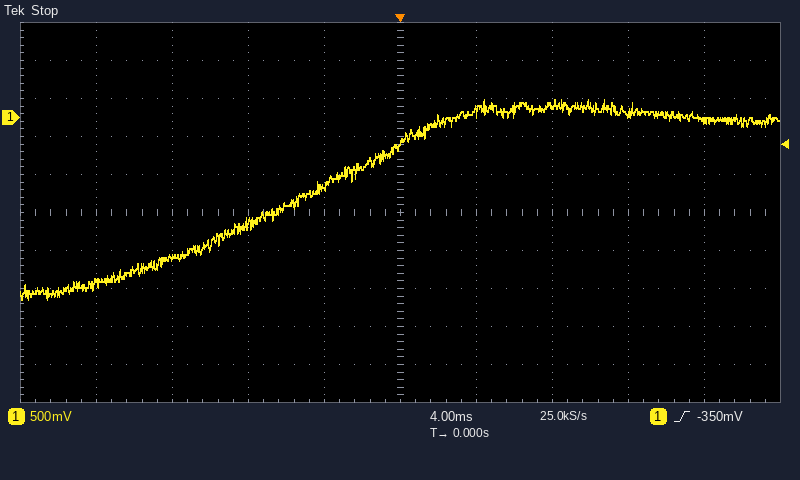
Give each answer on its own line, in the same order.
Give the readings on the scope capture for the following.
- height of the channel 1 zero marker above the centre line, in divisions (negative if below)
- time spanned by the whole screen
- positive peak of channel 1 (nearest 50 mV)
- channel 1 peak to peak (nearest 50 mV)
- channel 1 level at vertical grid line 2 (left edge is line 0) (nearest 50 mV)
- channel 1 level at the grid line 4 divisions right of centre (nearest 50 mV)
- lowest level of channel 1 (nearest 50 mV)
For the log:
+2.5 div
40 ms
250 mV
2.65 V
-1.85 V
-50 mV
-2.40 V
